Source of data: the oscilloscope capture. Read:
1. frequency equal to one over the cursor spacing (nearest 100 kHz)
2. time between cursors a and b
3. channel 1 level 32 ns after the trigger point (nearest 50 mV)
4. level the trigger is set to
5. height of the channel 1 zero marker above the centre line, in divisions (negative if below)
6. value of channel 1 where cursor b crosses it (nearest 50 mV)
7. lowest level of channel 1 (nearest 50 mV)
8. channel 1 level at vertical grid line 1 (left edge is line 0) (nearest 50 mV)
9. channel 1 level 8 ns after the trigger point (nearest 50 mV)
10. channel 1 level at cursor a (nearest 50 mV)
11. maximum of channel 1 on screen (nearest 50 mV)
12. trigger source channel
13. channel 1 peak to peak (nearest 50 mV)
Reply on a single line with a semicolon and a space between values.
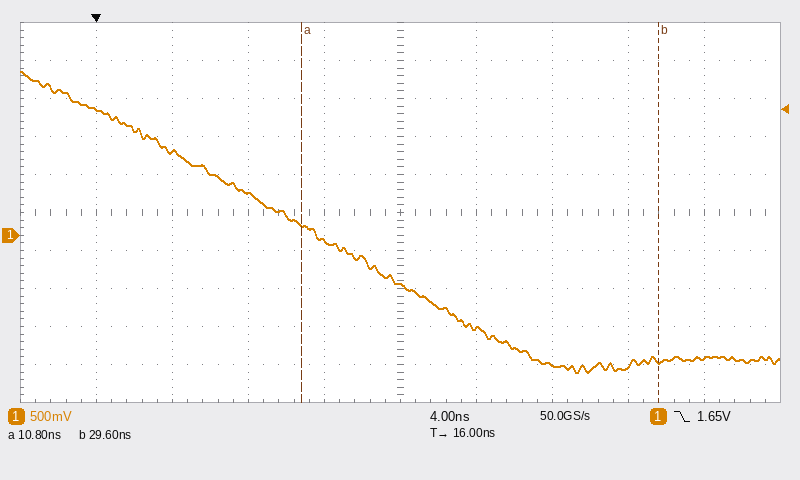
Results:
53.2 MHz; 18.8 ns; -1.60 V; 1.65 V; -0.6 div; -1.65 V; -1.80 V; 1.65 V; 550 mV; 150 mV; 2.15 V; channel 1; 3.95 V
